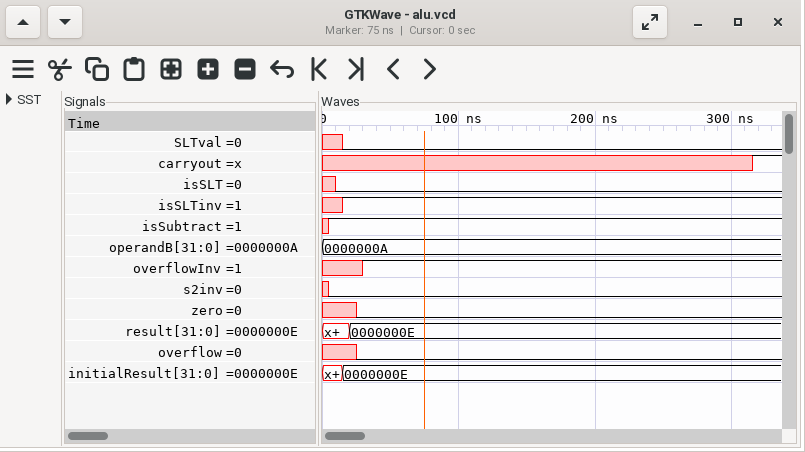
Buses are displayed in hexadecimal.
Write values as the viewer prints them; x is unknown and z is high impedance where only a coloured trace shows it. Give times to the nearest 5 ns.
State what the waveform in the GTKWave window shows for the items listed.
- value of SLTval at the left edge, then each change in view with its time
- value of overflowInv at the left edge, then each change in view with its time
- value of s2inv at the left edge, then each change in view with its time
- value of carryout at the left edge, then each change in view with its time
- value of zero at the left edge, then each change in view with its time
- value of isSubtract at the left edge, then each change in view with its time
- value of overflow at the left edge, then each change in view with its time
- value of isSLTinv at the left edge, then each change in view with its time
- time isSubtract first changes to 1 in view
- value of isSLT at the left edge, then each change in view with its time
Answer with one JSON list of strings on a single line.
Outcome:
["x, 0 at 15 ns", "x, 1 at 30 ns", "x, 0 at 5 ns", "x, 1 at 315 ns", "x, 0 at 25 ns", "x, 1 at 5 ns", "x, 0 at 25 ns", "x, 1 at 15 ns", "5 ns", "x, 0 at 10 ns"]
